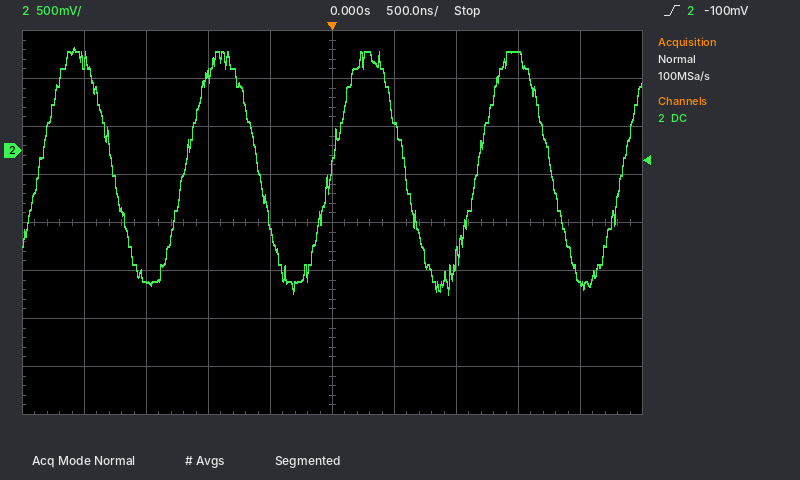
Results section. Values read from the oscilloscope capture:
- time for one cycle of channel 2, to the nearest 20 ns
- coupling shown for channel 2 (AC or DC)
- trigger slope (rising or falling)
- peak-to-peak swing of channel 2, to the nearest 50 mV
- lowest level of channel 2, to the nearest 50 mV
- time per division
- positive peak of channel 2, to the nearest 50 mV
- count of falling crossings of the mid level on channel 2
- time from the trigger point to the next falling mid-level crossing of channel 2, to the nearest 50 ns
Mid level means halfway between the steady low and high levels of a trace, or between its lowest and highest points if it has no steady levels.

1.18 µs
DC
rising
2.55 V
-1.50 V
500 ns
1.05 V
4
600 ns
